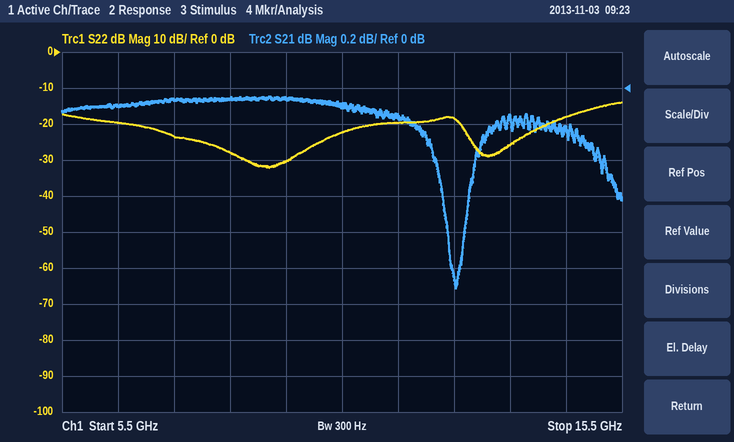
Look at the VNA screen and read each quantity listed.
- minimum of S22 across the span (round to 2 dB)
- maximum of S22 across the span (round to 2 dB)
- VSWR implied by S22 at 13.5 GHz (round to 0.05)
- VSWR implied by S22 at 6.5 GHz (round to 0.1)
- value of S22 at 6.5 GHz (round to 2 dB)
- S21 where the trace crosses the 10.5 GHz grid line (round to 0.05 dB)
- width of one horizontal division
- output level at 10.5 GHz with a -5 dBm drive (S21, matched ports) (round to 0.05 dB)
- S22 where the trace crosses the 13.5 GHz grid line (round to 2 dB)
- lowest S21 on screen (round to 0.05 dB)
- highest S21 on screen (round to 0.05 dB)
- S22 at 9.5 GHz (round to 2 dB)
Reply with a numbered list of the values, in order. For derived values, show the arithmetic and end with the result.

1. -32 dB
2. -14 dB
3. |Γ| = 10^(-26/20) = 0.0501; VSWR = (1 + 0.0501)/(1 − 0.0501) ≈ 1.11, so 1.10 to the nearest 0.05
4. |Γ| = 10^(-20/20) = 0.1000; VSWR = (1 + 0.1000)/(1 − 0.1000) ≈ 1.2
5. -20 dB
6. -0.10 dB
7. 1 GHz
8. -5 dBm + (-0.10 dB) = -5.10 dBm
9. -26 dB
10. -1.10 dB
11. -0.05 dB
12. -30 dB
